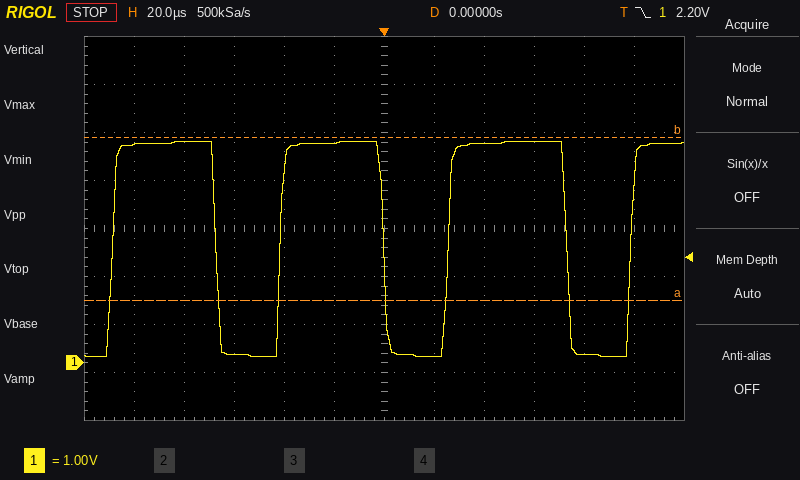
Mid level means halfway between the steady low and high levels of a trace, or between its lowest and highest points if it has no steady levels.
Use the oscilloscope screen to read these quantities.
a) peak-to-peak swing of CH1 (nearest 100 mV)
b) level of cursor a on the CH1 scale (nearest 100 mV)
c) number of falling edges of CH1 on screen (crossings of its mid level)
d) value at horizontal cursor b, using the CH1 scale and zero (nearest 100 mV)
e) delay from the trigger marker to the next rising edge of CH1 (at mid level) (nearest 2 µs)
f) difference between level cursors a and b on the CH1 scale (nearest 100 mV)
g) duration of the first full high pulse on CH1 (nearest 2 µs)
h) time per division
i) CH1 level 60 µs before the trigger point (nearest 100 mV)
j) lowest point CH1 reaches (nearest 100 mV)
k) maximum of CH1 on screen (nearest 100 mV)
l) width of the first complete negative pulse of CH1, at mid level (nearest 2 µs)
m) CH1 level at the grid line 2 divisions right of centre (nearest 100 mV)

4.5 V
1.3 V
3
4.7 V
26 µs
3.4 V
42 µs
20 µs
200 mV
100 mV
4.6 V
26 µs
4.6 V
